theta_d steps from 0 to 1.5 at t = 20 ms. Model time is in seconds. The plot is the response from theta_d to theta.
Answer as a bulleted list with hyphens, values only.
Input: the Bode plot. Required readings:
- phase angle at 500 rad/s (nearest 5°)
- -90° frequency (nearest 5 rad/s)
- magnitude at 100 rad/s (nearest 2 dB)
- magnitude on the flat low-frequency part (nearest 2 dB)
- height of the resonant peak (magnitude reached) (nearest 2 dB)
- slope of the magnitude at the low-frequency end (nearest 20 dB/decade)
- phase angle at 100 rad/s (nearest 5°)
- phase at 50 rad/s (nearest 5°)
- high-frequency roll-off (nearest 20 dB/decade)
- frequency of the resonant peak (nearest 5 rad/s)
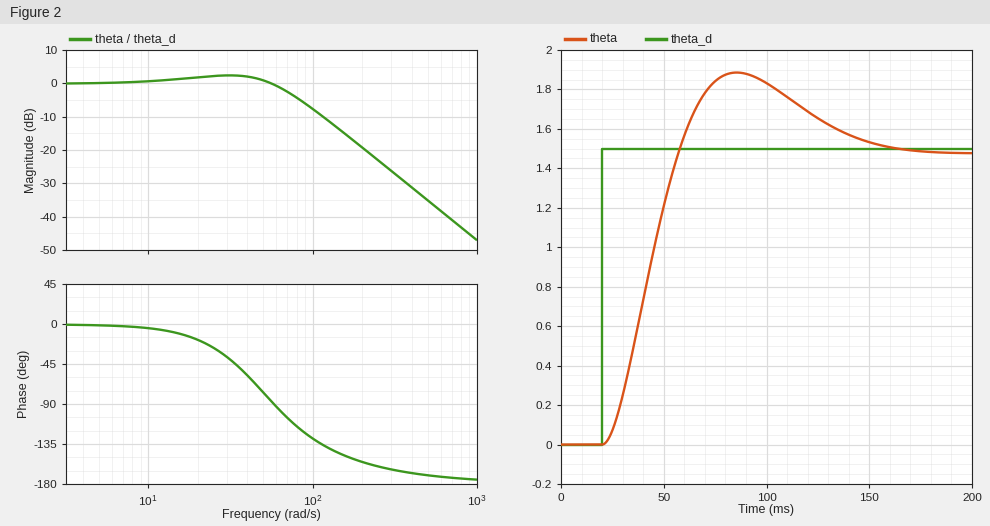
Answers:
- -170°
- 60 rad/s
- -8 dB
- 0 dB
- 2 dB
- 0 dB/decade
- -130°
- -75°
- -40 dB/decade
- 30 rad/s
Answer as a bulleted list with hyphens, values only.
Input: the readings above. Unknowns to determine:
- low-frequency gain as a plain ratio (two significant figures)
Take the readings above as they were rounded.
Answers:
- 1.0
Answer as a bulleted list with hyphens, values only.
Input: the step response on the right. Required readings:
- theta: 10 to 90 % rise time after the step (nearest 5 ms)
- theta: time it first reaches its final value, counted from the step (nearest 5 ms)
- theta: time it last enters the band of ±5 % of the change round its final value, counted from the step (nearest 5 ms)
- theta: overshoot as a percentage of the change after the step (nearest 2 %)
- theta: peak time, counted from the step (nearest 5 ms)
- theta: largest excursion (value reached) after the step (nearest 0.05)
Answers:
- 25 ms
- 35 ms
- 125 ms
- 28 %
- 65 ms
- 1.90
